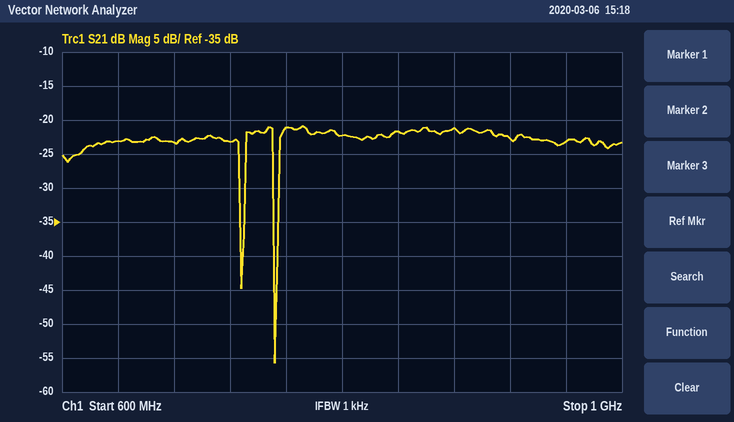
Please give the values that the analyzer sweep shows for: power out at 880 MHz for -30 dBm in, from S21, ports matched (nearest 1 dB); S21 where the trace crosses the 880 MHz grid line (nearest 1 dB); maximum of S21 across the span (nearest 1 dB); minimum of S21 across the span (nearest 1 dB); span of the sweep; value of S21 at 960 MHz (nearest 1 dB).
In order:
-51 dBm
-21 dB
-21 dB
-56 dB
400 MHz
-23 dB
